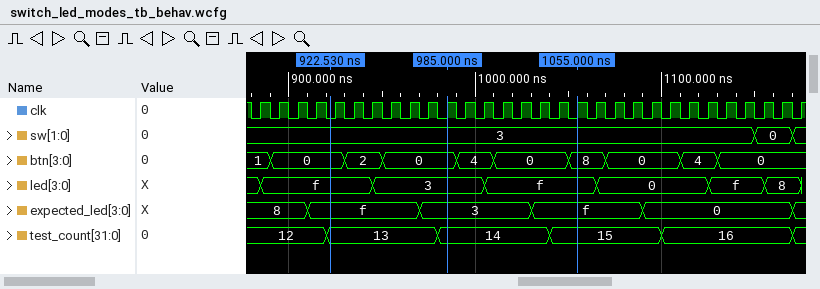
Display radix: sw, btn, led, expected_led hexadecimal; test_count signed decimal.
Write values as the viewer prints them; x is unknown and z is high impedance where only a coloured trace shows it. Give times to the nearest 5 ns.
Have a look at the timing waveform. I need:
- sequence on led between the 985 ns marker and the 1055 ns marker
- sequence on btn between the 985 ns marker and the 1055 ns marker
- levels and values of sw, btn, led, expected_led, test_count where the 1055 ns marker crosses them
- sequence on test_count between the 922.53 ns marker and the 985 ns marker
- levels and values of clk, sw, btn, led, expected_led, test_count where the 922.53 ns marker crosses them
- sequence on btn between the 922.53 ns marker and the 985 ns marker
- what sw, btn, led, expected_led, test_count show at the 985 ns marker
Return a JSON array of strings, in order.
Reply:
["3, f", "0, 4, 0, 8", "sw=3, btn=8, led=f, expected_led=f, test_count=15", "13, 14", "clk=0, sw=3, btn=0, led=f, expected_led=f, test_count=13", "0, 2, 0", "sw=3, btn=0, led=3, expected_led=3, test_count=14"]
